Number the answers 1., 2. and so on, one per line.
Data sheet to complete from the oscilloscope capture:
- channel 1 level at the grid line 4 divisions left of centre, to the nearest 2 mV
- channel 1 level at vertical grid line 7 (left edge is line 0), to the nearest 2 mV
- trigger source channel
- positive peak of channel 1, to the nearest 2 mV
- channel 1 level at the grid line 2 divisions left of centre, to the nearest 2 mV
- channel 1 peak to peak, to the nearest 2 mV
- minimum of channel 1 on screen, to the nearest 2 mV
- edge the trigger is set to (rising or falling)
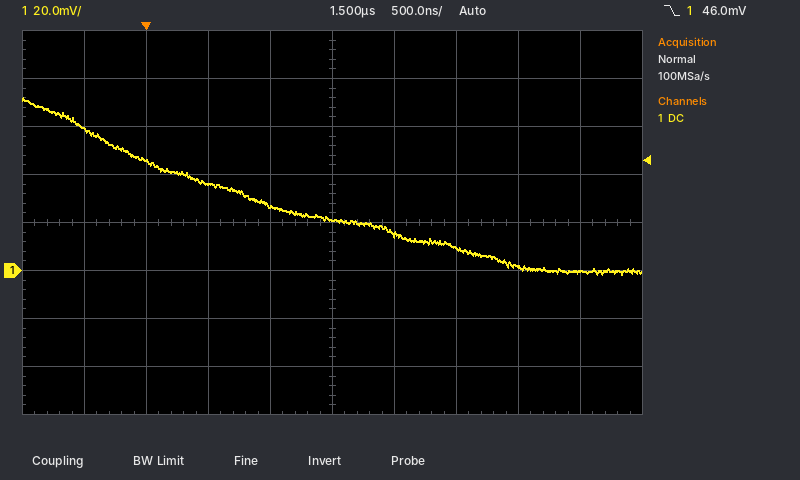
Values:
1. 58 mV
2. 10 mV
3. channel 1
4. 72 mV
5. 36 mV
6. 74 mV
7. -2 mV
8. falling
